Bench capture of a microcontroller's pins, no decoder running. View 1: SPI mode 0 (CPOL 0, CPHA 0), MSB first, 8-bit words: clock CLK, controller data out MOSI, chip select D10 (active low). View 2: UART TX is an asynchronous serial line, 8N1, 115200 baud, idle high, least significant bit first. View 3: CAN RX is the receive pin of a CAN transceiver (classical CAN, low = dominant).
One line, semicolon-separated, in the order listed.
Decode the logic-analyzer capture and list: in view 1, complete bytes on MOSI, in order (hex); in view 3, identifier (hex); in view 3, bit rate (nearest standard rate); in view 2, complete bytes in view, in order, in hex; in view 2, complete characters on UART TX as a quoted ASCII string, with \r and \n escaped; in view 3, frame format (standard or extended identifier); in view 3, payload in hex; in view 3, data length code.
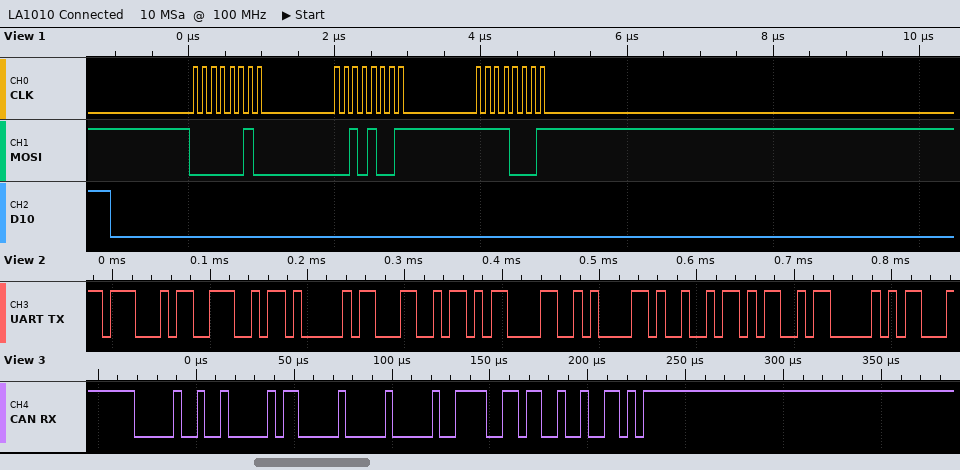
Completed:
02 29 F1; 0x012; 250 kbit/s; 47 4E 41 4C 0D 0A 49 4D 50; "GNAL\r\nIMP"; standard; 00 00 79; 3
